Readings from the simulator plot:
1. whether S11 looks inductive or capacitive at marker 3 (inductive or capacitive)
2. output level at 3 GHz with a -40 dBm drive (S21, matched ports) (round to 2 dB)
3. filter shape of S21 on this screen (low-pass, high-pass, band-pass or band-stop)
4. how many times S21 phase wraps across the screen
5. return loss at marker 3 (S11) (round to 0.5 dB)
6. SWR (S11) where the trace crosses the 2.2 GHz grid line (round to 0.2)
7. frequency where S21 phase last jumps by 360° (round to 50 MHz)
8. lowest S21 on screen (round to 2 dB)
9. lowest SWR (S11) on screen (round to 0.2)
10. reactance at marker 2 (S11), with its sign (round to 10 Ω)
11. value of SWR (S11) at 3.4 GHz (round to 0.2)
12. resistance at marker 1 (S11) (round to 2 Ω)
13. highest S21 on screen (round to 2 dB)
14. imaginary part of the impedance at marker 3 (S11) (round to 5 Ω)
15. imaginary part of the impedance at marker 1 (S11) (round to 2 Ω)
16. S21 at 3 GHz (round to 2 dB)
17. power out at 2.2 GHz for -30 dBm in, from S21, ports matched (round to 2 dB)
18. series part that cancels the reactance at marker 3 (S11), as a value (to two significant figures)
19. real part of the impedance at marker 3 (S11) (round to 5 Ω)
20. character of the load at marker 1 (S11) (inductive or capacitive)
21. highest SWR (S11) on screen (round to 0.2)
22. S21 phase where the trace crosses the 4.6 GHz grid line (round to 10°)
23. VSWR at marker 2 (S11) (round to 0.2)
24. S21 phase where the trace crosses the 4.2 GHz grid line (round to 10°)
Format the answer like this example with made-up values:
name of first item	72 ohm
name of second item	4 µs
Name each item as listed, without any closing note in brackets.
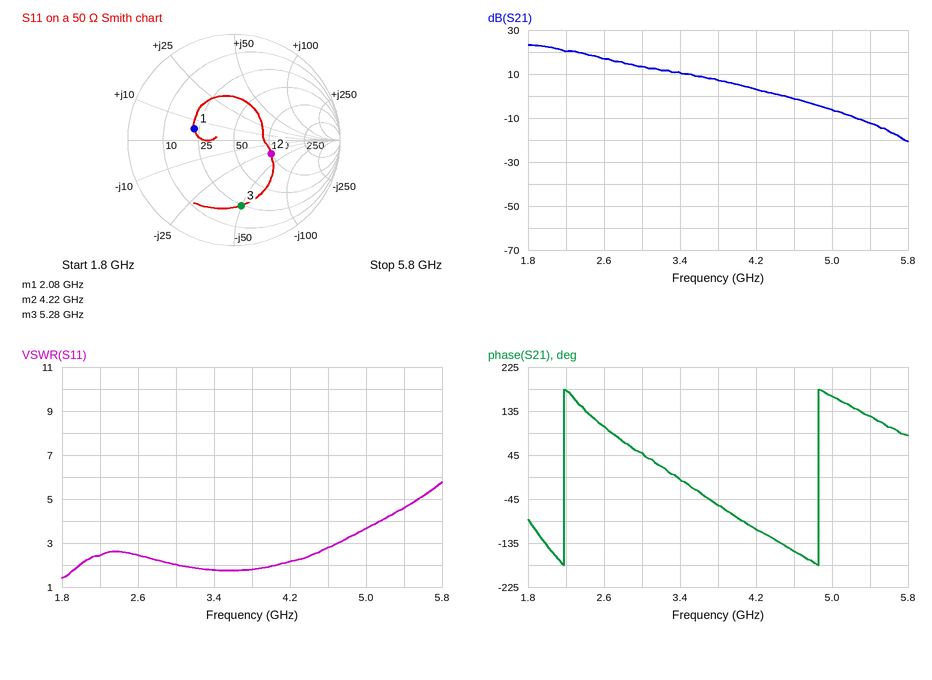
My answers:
whether S11 looks inductive or capacitive at marker 3	capacitive
output level at 3 GHz with a -40 dBm drive (S21, matched ports)	-26 dBm
filter shape of S21 on this screen	low-pass
how many times S21 phase wraps across the screen	2
return loss at marker 3 (S11)	4.0 dB
SWR (S11) where the trace crosses the 2.2 GHz grid line	2.4
frequency where S21 phase last jumps by 360°	4.85 GHz
lowest S21 on screen	-20 dB
lowest SWR (S11) on screen	1.4
reactance at marker 2 (S11), with its sign	-30 Ω
value of SWR (S11) at 3.4 GHz	1.8
resistance at marker 1 (S11)	22 Ω
highest S21 on screen	24 dB
imaginary part of the impedance at marker 3 (S11)	-50 Ω
imaginary part of the impedance at marker 1 (S11)	+6 Ω
S21 at 3 GHz	14 dB
power out at 2.2 GHz for -30 dBm in, from S21, ports matched	-10 dBm
series part that cancels the reactance at marker 3 (S11), as a value	1.5 nH
real part of the impedance at marker 3 (S11)	25 Ω
character of the load at marker 1 (S11)	inductive
highest SWR (S11) on screen	5.8
S21 phase where the trace crosses the 4.6 GHz grid line	-150°
VSWR at marker 2 (S11)	2.2
S21 phase where the trace crosses the 4.2 GHz grid line	-110°
